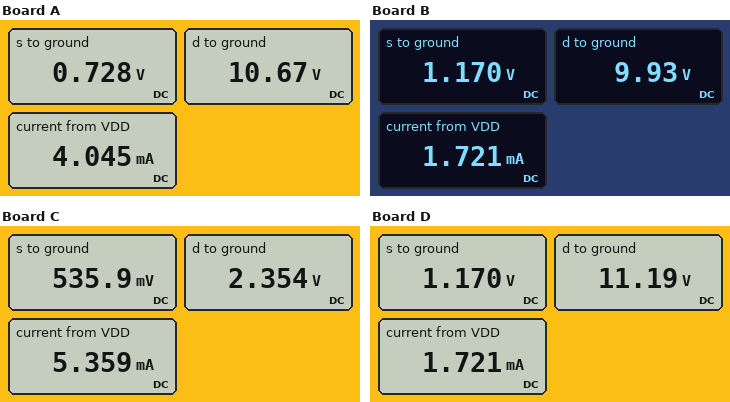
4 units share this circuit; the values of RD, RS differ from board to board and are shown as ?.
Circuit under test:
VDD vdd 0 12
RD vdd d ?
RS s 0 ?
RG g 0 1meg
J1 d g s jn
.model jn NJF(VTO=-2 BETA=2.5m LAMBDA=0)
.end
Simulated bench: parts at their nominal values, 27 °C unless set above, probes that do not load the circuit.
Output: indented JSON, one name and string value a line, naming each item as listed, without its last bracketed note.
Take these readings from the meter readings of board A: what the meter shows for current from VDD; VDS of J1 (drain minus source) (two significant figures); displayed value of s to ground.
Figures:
{
  "what the meter shows for current from VDD": "4.045 mA",
  "VDS of J1 (drain minus source)": "9.9 V",
  "displayed value of s to ground": "0.728 V"
}
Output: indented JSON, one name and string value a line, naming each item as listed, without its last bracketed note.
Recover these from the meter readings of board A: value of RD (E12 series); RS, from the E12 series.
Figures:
{
  "value of RD": "330 Ω",
  "RS, from the E12 series": "180 Ω"
}
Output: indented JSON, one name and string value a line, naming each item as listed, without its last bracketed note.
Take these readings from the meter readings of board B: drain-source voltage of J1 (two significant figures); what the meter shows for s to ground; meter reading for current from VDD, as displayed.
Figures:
{
  "drain-source voltage of J1": "8.8 V",
  "what the meter shows for s to ground": "1.170 V",
  "meter reading for current from VDD, as displayed": "1.721 mA"
}
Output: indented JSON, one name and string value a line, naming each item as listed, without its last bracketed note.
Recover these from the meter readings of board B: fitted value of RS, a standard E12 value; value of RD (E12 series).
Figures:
{
  "fitted value of RS, a standard E12 value": "680 Ω",
  "value of RD": "1.2 kΩ"
}
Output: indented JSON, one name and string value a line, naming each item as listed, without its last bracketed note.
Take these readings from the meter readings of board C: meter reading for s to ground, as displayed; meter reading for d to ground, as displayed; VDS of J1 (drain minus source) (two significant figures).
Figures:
{
  "meter reading for s to ground, as displayed": "535.9 mV",
  "meter reading for d to ground, as displayed": "2.354 V",
  "VDS of J1 (drain minus source)": "1.8 V"
}
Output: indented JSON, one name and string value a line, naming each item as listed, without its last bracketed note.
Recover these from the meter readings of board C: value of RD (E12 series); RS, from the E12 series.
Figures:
{
  "value of RD": "1.8 kΩ",
  "RS, from the E12 series": "100 Ω"
}
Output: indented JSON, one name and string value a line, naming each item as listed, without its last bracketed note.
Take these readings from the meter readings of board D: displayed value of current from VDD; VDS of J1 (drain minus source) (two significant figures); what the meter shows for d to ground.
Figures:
{
  "displayed value of current from VDD": "1.721 mA",
  "VDS of J1 (drain minus source)": "10 V",
  "what the meter shows for d to ground": "11.19 V"
}
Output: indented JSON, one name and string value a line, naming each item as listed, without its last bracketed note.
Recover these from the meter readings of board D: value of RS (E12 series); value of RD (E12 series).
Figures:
{
  "value of RS": "680 Ω",
  "value of RD": "470 Ω"
}
